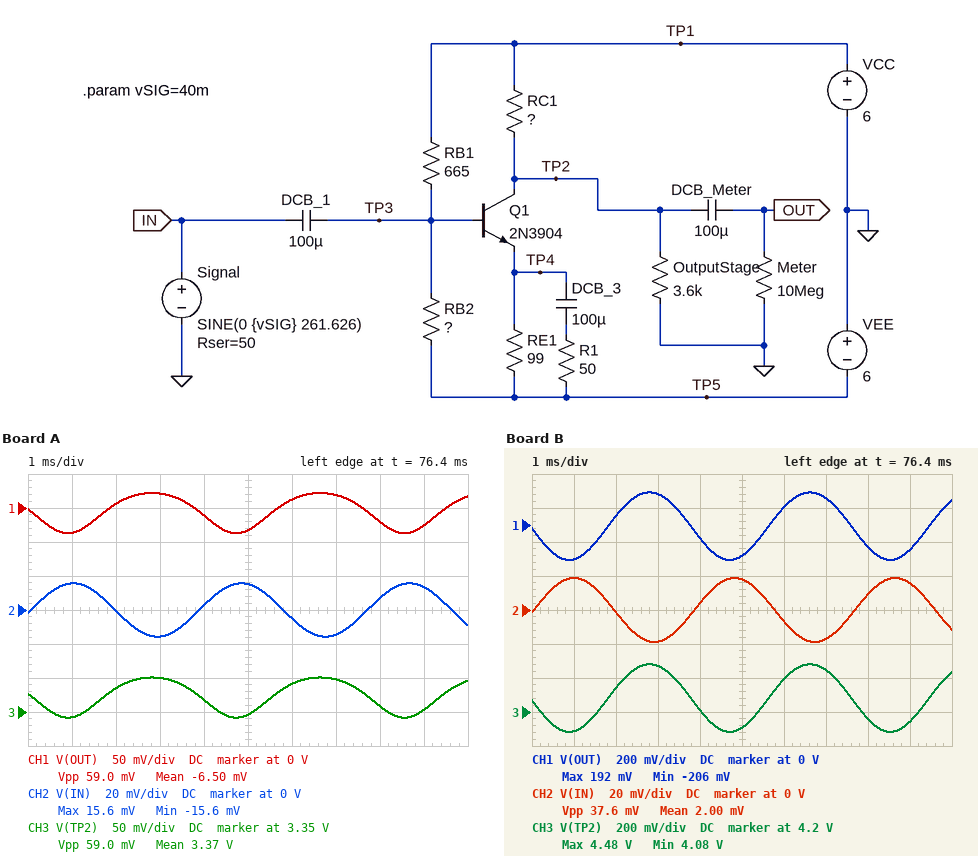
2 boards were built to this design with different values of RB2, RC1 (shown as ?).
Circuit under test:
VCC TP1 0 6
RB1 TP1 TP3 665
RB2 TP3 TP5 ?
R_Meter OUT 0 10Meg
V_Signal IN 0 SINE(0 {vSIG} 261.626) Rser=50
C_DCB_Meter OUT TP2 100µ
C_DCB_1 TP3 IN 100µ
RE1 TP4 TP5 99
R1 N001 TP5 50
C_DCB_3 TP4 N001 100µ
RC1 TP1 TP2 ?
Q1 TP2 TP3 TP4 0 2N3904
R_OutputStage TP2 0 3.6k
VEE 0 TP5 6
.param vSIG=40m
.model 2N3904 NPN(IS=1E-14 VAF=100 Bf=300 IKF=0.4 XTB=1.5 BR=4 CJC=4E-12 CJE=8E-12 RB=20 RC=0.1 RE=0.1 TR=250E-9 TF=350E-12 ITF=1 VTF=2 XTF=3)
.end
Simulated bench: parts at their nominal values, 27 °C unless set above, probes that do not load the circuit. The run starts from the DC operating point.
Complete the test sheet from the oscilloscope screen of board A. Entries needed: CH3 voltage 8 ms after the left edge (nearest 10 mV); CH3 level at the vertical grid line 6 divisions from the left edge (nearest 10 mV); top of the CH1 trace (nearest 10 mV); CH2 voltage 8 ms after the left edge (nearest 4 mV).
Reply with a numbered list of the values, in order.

1. 3.36 V
2. 3.39 V
3. 20 mV
4. 8 mV
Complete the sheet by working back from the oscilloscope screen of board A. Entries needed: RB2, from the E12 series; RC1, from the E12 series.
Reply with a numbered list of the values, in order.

1. 33 Ω
2. 2.7 kΩ
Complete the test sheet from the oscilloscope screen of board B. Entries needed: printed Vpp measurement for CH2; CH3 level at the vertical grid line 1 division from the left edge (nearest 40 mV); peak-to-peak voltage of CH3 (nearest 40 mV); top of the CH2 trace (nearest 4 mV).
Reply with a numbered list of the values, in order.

1. 37.6 mV
2. 4.08 V
3. 400 mV
4. 20 mV
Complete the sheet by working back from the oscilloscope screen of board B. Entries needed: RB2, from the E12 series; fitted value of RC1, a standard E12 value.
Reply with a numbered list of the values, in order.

1. 47 Ω
2. 680 Ω
